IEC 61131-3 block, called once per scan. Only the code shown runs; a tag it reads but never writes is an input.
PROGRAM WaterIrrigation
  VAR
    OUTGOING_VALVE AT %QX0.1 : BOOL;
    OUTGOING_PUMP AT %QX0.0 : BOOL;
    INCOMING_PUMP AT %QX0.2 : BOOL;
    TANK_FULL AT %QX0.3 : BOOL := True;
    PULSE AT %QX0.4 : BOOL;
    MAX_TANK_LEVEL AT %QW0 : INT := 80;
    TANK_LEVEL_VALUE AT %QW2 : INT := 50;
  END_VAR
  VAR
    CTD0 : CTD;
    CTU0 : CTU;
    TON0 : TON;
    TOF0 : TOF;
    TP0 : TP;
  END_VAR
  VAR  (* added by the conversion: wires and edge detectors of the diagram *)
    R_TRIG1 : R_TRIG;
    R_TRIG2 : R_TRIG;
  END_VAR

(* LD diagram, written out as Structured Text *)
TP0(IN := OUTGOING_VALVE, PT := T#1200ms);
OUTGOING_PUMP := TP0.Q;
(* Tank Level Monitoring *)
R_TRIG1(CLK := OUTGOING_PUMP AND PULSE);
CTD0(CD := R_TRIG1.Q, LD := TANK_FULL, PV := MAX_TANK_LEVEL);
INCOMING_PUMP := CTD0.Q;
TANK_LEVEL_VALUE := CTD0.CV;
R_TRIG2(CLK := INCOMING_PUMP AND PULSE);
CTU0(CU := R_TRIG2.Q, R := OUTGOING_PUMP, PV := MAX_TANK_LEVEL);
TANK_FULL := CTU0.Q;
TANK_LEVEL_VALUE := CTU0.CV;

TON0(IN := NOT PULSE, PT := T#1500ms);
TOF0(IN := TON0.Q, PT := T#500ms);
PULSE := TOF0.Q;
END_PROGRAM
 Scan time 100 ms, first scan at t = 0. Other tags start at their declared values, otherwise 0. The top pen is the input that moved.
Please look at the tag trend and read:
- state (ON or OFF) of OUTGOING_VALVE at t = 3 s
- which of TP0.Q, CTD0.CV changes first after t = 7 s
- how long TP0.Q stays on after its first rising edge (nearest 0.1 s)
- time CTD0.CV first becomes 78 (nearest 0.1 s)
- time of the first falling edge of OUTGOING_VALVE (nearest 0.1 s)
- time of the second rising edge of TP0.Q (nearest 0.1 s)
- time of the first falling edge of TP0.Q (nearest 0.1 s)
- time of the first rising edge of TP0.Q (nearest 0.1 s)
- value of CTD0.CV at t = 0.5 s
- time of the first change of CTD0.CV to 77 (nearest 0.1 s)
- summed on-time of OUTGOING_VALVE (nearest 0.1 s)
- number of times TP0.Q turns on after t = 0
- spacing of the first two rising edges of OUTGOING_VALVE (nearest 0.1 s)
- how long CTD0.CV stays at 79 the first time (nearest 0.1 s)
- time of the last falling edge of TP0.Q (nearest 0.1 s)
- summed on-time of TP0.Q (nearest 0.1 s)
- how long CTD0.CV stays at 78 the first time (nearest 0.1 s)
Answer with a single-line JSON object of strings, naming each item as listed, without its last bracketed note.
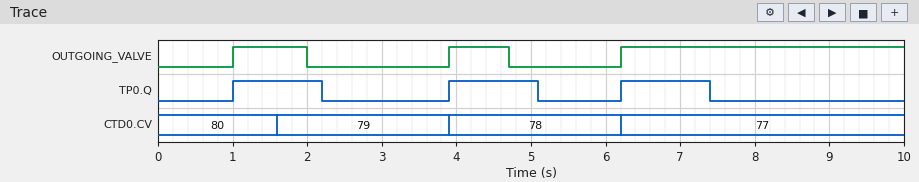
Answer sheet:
{"state (ON or OFF) of OUTGOING_VALVE at t = 3 s": "OFF", "which of TP0.Q, CTD0.CV changes first after t = 7 s": "TP0.Q", "how long TP0.Q stays on after its first rising edge": "1.2 s", "time CTD0.CV first becomes 78": "3.9 s", "time of the first falling edge of OUTGOING_VALVE": "2.0 s", "time of the second rising edge of TP0.Q": "3.9 s", "time of the first falling edge of TP0.Q": "2.2 s", "time of the first rising edge of TP0.Q": "1.0 s", "value of CTD0.CV at t = 0.5 s": "80", "time of the first change of CTD0.CV to 77": "6.2 s", "summed on-time of OUTGOING_VALVE": "5.6 s", "number of times TP0.Q turns on after t = 0": "3", "spacing of the first two rising edges of OUTGOING_VALVE": "2.9 s", "how long CTD0.CV stays at 79 the first time": "2.3 s", "time of the last falling edge of TP0.Q": "7.4 s", "summed on-time of TP0.Q": "3.6 s", "how long CTD0.CV stays at 78 the first time": "2.3 s"}
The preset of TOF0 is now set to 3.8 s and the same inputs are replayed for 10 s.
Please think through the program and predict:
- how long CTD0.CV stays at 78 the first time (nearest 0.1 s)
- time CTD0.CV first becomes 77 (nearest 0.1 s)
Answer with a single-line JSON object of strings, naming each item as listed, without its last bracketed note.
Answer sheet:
{"how long CTD0.CV stays at 78 the first time": "3.2 s", "time CTD0.CV first becomes 77": "7.1 s"}
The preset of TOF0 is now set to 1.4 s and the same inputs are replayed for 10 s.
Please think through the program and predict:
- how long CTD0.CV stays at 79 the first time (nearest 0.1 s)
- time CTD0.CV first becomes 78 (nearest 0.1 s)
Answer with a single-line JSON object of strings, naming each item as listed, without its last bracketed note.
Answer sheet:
{"how long CTD0.CV stays at 79 the first time": "3.1 s", "time CTD0.CV first becomes 78": "4.7 s"}
